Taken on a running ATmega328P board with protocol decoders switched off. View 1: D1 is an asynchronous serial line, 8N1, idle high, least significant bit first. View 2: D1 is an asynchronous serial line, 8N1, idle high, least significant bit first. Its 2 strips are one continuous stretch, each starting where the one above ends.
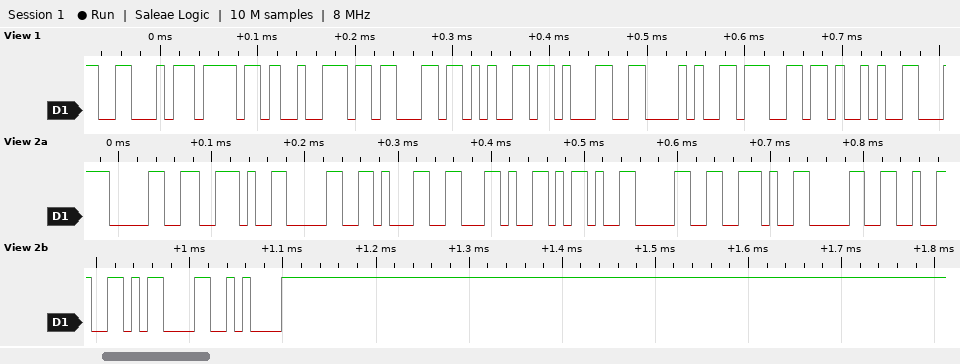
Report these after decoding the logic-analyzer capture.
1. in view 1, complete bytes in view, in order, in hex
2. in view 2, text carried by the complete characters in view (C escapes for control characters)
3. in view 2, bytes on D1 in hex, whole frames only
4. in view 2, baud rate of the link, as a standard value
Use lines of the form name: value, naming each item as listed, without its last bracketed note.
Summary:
in view 1, complete bytes in view, in order, in hex: 46 6F 72 63 65 31 28 67 29
in view 2, text carried by the complete characters in view: "0.01,-0.02\r\n"
in view 2, bytes on D1 in hex, whole frames only: 30 2E 30 31 2C 2D 30 2E 30 32 0D 0A
in view 2, baud rate of the link, as a standard value: 115200 baud
